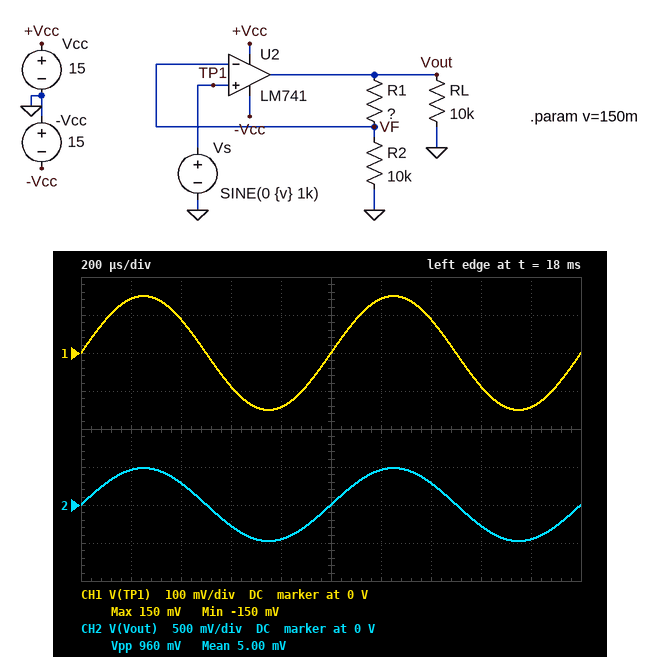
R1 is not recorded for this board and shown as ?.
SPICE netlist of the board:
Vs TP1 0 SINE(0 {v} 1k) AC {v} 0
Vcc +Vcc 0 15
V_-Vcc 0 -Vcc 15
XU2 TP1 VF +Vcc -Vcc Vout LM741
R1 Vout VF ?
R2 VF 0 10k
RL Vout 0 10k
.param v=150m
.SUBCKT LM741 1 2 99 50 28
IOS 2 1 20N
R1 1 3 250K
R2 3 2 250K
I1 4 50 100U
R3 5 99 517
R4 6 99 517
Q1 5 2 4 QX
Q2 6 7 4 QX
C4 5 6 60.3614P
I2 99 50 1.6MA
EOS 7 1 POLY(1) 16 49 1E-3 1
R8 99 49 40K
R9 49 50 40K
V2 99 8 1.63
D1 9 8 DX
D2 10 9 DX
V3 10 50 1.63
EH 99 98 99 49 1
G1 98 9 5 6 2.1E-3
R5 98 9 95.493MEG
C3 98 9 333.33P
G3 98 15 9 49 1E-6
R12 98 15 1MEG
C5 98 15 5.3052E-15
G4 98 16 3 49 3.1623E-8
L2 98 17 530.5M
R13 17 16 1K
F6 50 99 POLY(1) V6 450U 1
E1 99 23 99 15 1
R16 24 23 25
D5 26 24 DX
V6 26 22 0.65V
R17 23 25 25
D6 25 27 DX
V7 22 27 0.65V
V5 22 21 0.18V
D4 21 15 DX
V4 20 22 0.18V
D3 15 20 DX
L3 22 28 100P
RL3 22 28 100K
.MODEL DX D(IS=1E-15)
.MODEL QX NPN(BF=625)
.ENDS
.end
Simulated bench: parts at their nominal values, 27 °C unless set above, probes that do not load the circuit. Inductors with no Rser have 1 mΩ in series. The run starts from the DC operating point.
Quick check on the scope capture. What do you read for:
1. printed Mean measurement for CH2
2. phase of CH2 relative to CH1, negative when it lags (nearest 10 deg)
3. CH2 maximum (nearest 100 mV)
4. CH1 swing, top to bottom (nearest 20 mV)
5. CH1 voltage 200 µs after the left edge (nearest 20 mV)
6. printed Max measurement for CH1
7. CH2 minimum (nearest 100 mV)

5.00 mV
0 deg
500 mV
300 mV
140 mV
150 mV
-500 mV
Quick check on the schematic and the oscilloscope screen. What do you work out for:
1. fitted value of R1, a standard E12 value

22 kΩ
